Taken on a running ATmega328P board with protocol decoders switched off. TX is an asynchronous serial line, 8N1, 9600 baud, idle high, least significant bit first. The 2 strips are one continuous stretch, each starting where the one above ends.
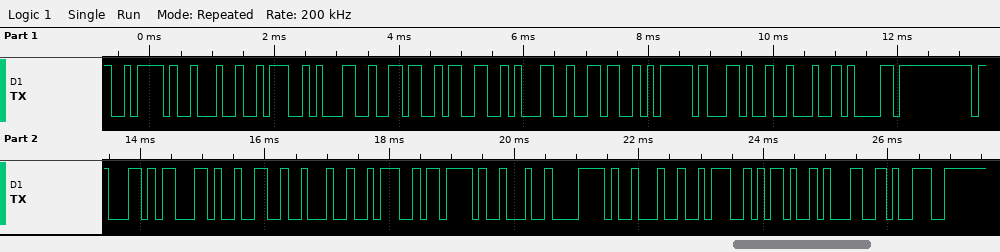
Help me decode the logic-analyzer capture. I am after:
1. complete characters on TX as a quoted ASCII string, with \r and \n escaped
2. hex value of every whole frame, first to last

"z\":16316},\"acc2\":{\"x\":-19"
7A 22 3A 31 36 33 31 36 7D 2C 22 61 63 63 32 22 3A 7B 22 78 22 3A 2D 31 39
